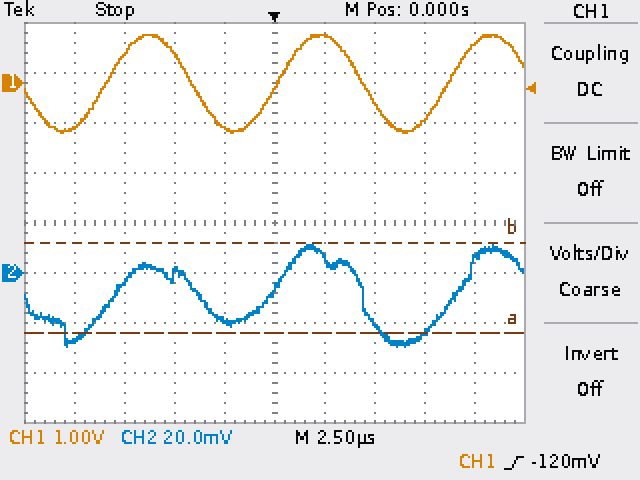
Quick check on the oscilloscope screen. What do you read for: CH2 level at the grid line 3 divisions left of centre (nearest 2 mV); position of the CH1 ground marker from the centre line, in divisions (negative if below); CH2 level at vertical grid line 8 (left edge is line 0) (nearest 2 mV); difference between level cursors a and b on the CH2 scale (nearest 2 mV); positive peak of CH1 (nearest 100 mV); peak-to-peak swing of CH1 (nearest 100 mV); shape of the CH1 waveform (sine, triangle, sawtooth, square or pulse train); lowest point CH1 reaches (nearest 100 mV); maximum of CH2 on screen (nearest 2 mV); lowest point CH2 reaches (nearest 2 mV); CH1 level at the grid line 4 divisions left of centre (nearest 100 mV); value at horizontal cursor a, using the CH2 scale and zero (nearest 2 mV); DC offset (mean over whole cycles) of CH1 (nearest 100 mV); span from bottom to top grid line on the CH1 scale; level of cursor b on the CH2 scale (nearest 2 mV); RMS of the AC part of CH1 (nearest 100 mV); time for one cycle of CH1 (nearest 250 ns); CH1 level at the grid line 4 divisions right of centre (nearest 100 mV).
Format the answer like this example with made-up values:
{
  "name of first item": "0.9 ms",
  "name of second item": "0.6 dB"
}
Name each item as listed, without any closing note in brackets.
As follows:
{
  "CH2 level at the grid line 3 divisions left of centre": "-4 mV",
  "position of the CH1 ground marker from the centre line, in divisions": "+2.8 div",
  "CH2 level at vertical grid line 8 (left edge is line 0)": "-24 mV",
  "difference between level cursors a and b on the CH2 scale": "36 mV",
  "positive peak of CH1": "1.0 V",
  "peak-to-peak swing of CH1": "2.0 V",
  "shape of the CH1 waveform": "sine",
  "lowest point CH1 reaches": "-1.0 V",
  "maximum of CH2 on screen": "12 mV",
  "lowest point CH2 reaches": "-30 mV",
  "CH1 level at the grid line 4 divisions left of centre": "-900 mV",
  "value at horizontal cursor a, using the CH2 scale and zero": "-24 mV",
  "DC offset (mean over whole cycles) of CH1": "0.0 V",
  "span from bottom to top grid line on the CH1 scale": "8 V",
  "level of cursor b on the CH2 scale": "12 mV",
  "RMS of the AC part of CH1": "700 mV",
  "time for one cycle of CH1": "8.50 µs",
  "CH1 level at the grid line 4 divisions right of centre": "800 mV"
}
